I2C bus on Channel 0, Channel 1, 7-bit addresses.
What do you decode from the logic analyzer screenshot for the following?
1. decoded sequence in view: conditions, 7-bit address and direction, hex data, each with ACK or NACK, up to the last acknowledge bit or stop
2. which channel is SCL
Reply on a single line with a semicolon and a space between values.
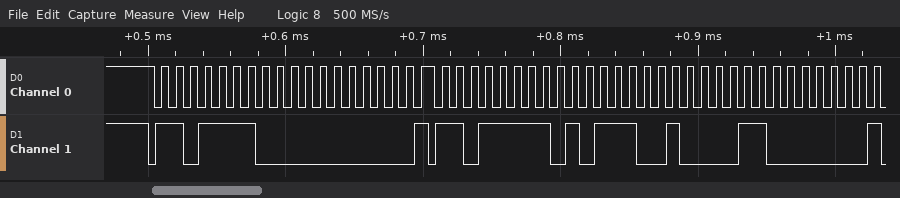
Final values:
start, address 6F write ACK, 00 ACK, repeated start, address 6F read ACK, B9 ACK, 18 ACK; Channel 0
